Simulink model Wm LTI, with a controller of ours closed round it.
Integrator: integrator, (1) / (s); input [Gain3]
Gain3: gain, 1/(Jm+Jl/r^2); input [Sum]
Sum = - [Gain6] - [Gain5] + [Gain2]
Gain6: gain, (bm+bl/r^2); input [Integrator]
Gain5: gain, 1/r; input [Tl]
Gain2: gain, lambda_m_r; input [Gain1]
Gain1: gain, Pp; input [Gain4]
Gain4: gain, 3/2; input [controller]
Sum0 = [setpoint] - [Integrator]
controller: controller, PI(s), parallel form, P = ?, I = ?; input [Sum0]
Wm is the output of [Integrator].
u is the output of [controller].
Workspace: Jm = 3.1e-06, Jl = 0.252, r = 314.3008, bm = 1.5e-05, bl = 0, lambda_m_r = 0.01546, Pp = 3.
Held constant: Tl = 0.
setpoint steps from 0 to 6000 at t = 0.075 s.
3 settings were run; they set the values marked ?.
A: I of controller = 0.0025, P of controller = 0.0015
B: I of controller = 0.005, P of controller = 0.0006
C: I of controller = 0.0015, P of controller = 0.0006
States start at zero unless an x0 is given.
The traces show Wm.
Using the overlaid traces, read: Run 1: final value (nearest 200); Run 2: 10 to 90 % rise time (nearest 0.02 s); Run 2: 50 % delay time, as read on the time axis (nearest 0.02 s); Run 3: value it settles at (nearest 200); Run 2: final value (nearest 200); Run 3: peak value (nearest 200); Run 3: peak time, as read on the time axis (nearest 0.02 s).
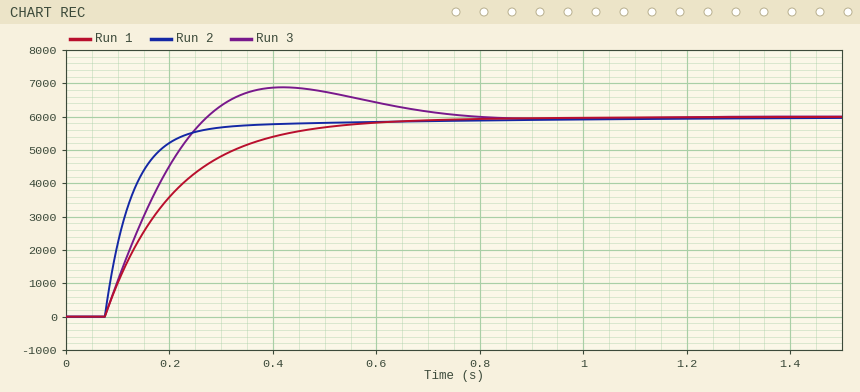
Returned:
6000
0.14 s
0.12 s
6000
6000
6800
0.42 s
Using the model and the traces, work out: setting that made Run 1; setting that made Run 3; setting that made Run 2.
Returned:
C
B
A
